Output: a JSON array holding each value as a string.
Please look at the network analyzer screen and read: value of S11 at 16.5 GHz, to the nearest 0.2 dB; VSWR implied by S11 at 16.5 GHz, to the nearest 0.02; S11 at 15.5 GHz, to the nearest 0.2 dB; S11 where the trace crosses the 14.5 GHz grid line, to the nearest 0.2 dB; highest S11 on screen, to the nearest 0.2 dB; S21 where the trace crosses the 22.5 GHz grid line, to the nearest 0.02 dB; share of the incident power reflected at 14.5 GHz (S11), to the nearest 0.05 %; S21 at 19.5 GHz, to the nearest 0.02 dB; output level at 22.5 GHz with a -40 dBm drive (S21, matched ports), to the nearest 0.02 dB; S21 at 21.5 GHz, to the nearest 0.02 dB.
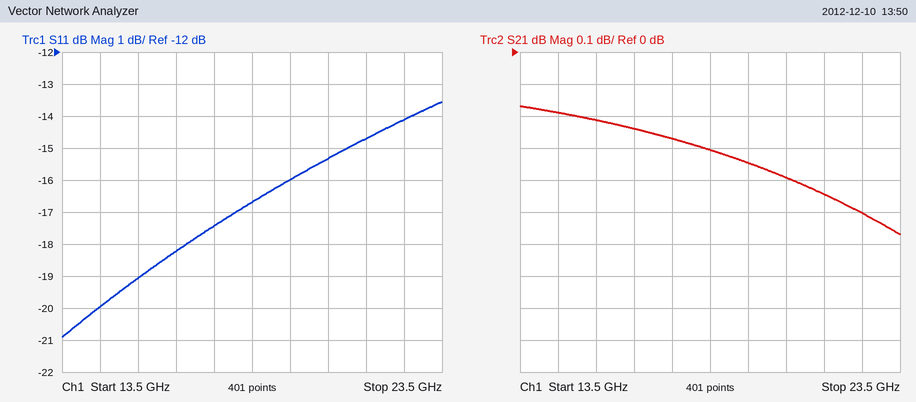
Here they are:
["-18.2 dB", "1.28", "-19.0 dB", "-20.0 dB", "-13.6 dB", "-0.50 dB", "1.00 %", "-0.34 dB", "-40.50 dBm", "-0.44 dB"]
